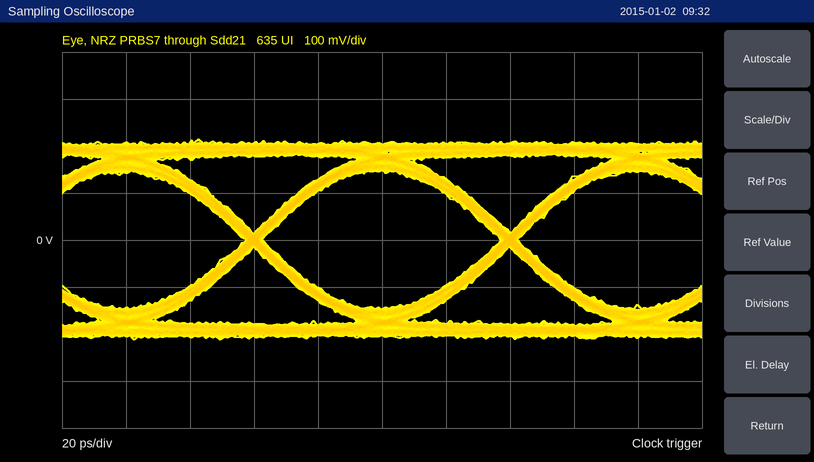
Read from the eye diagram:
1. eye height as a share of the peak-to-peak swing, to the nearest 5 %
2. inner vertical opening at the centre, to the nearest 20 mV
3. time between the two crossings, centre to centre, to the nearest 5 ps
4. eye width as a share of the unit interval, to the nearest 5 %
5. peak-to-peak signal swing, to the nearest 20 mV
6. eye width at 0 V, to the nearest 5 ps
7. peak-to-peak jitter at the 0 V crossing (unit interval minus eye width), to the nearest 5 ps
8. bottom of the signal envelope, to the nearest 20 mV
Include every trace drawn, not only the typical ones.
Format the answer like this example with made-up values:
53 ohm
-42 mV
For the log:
70 %
300 mV
80 ps
95 %
420 mV
75 ps
5 ps
-220 mV
